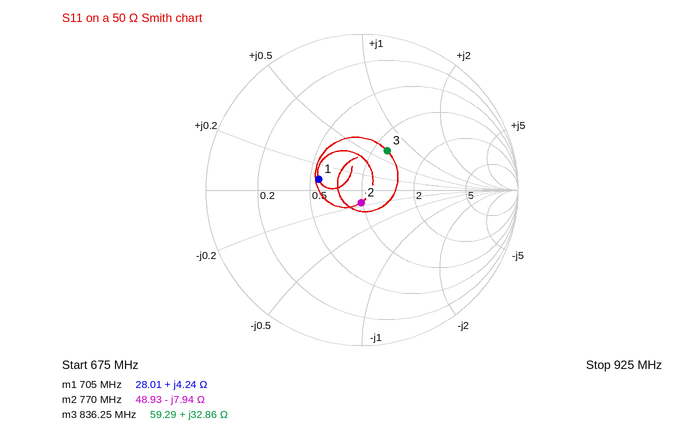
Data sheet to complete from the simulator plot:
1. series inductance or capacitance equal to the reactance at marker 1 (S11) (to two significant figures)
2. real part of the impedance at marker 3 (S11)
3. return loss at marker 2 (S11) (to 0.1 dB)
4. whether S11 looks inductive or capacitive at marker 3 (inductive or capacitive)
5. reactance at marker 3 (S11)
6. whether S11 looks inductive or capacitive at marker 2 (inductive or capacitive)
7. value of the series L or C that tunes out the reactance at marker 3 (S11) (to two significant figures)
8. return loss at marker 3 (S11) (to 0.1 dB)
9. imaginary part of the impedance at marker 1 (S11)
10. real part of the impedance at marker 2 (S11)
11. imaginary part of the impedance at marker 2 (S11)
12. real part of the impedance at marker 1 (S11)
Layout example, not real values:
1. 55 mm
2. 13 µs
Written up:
1. 960 pH
2. 59.29 Ω
3. 21.9 dB
4. inductive
5. +32.86 Ω
6. capacitive
7. 5.8 pF
8. 10.5 dB
9. +4.24 Ω
10. 48.93 Ω
11. -7.94 Ω
12. 28.01 Ω
